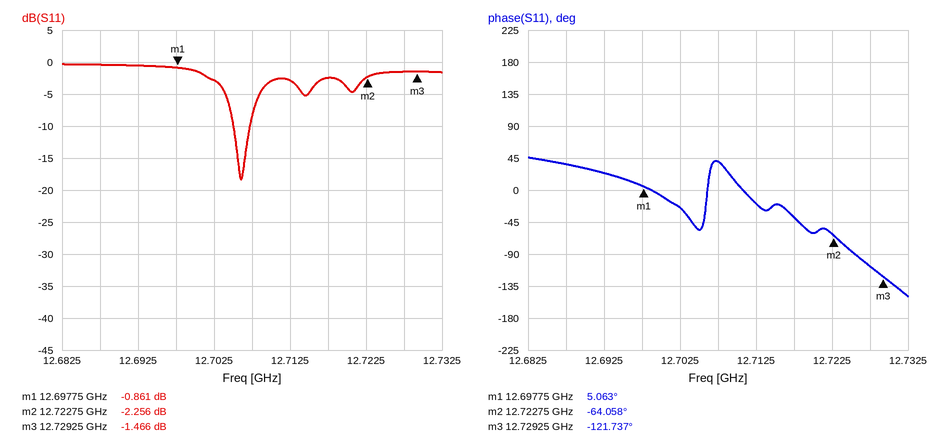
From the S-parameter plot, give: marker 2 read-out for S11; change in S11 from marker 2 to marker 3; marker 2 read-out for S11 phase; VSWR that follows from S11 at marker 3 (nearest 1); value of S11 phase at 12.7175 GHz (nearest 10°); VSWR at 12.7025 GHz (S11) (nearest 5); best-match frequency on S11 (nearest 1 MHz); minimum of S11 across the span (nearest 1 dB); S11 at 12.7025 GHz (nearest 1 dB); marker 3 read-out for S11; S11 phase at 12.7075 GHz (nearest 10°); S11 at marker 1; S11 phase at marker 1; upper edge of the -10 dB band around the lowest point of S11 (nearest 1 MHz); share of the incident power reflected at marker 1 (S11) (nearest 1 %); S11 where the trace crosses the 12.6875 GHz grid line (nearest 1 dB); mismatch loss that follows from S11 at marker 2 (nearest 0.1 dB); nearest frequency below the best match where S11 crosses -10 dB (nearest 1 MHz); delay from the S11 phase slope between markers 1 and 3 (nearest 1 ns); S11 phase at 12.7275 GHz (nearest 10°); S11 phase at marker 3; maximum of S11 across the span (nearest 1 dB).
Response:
-2.256 dB
0.790 dB
-64.058°
12
-40°
5
12.706 GHz
-18 dB
-3 dB
-1.466 dB
40°
-0.861 dB
5.063°
12.707 GHz
82 %
0 dB
3.9 dB
12.705 GHz
11 ns
-110°
-121.737°
0 dB
